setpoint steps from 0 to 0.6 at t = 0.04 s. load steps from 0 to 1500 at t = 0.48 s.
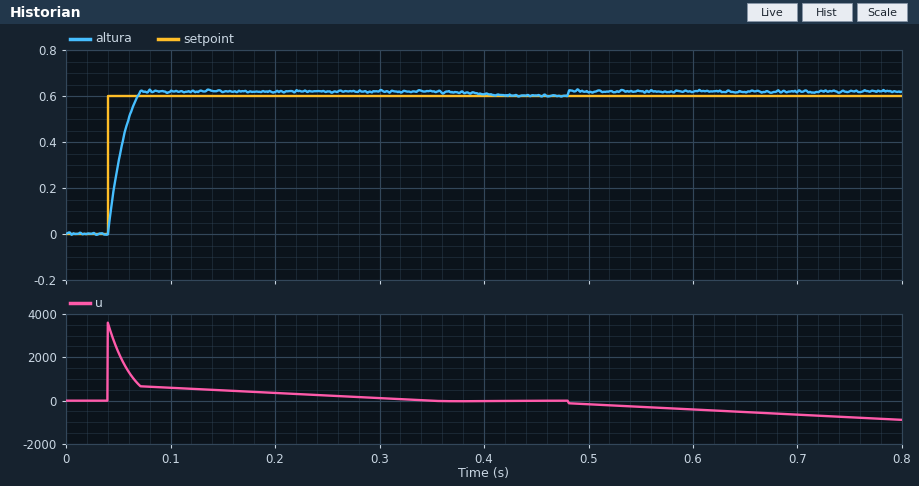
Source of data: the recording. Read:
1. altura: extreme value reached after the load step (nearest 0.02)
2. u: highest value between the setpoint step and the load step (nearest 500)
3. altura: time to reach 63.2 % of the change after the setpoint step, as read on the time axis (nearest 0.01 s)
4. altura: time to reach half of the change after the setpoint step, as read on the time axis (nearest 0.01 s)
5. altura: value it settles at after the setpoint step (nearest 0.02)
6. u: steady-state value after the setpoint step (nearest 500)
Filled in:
0.62
3500
0.05 s
0.05 s
0.60
0
